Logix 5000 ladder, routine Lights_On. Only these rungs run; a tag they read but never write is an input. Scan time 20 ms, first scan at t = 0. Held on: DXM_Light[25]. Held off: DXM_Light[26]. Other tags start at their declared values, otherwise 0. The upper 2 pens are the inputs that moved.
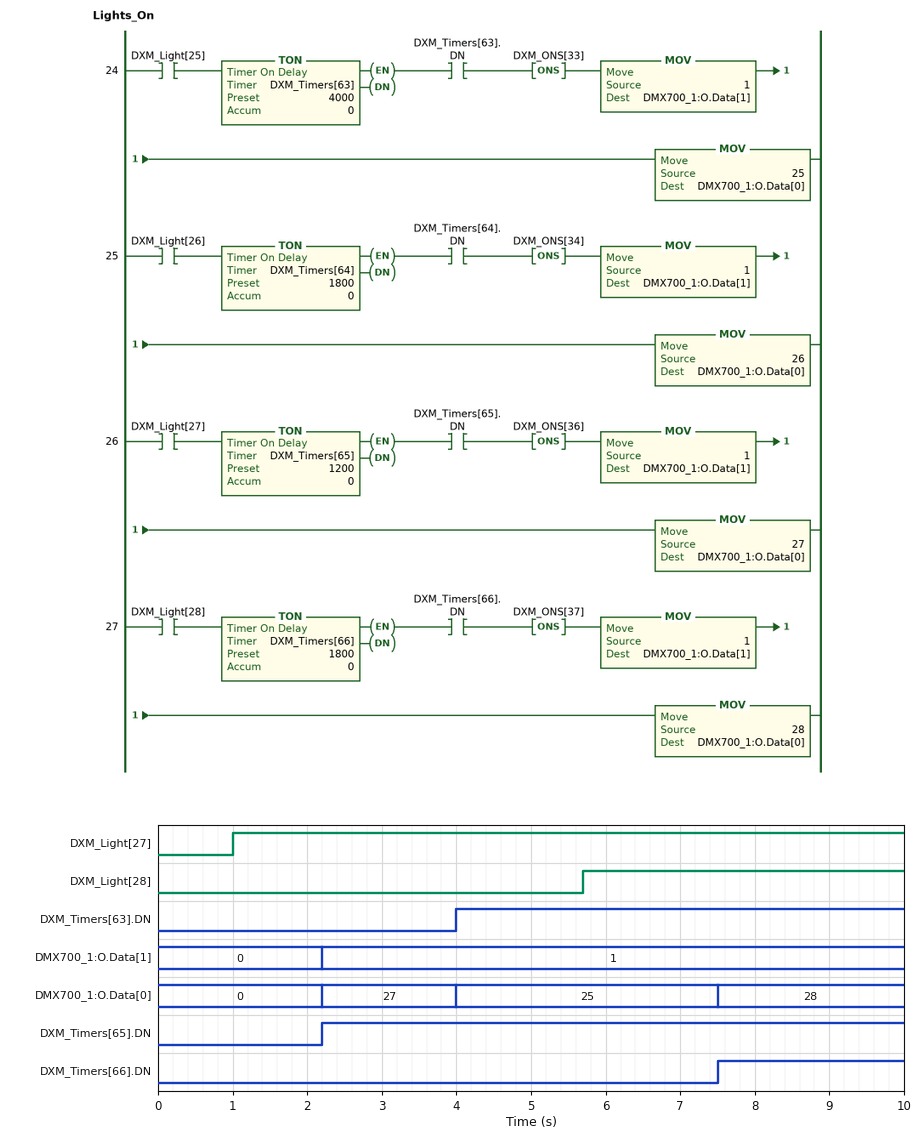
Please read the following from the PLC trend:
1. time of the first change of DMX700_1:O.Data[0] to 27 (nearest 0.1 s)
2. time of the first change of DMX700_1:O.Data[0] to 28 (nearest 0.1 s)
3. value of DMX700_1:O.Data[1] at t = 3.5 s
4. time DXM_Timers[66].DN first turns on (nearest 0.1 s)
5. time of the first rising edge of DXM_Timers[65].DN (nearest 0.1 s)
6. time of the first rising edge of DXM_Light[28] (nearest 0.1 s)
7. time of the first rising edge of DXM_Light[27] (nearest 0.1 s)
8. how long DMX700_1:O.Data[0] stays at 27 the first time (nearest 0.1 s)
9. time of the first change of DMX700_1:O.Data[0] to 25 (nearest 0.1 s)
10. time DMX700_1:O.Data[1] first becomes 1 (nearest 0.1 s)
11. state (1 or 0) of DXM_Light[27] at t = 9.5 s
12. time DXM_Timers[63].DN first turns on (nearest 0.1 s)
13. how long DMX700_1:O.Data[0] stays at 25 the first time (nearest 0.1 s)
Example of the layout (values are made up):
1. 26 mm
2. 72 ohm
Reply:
1. 2.2 s
2. 7.5 s
3. 1
4. 7.5 s
5. 2.2 s
6. 5.7 s
7. 1.0 s
8. 1.8 s
9. 4.0 s
10. 2.2 s
11. 1
12. 4.0 s
13. 3.5 s
